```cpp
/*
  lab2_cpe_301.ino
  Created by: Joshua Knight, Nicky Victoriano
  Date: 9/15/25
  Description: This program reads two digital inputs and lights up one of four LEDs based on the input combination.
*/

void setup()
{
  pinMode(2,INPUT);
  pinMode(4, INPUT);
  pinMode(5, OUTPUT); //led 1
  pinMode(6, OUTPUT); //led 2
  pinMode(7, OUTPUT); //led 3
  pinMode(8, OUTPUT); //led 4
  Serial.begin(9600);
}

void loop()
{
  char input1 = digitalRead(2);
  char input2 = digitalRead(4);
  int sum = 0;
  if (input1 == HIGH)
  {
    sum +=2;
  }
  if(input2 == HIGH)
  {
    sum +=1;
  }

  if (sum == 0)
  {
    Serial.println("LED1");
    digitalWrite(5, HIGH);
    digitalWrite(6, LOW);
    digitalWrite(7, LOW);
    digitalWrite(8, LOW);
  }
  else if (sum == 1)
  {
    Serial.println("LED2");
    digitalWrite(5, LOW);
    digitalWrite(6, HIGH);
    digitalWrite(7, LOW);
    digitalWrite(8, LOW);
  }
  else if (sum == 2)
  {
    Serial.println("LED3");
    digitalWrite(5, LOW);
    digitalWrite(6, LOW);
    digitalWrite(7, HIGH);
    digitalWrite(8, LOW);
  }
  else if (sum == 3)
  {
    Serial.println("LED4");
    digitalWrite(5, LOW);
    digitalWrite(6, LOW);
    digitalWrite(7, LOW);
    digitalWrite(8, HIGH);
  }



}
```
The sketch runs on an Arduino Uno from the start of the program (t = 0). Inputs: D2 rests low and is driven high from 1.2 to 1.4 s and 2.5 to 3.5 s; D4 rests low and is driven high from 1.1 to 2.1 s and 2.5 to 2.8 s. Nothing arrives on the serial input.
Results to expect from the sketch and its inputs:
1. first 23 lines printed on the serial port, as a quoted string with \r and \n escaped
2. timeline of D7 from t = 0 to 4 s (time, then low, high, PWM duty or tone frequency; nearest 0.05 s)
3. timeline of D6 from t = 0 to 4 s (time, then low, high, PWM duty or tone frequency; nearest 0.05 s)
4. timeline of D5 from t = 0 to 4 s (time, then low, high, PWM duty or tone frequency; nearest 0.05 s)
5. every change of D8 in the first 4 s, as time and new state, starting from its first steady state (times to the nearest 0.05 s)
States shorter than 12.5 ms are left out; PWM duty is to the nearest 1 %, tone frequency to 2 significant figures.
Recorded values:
"LED1\r\nLED1\r\nLED1\r\nLED1\r\nLED1\r\nLED1\r\nLED1\r\nLED1\r\nLED1\r\nLED1\r\nLED1\r\nLED1\r\nLED1\r\nLED1\r\nLED1\r\nLED1\r\nLED1\r\nLED1\r\nLED1\r\nLED1\r\nLED1\r\nLED1\r\nLED1\r\n"
0 s low; 2.8 s high; 3.5 s low
0 s low; 1.1 s high; 1.2 s low; 1.4 s high; 2.1 s low
0 s high; 1.1 s low; 2.1 s high; 2.5 s low; 3.5 s high
0 s low; 1.2 s high; 1.4 s low; 2.5 s high; 2.8 s low
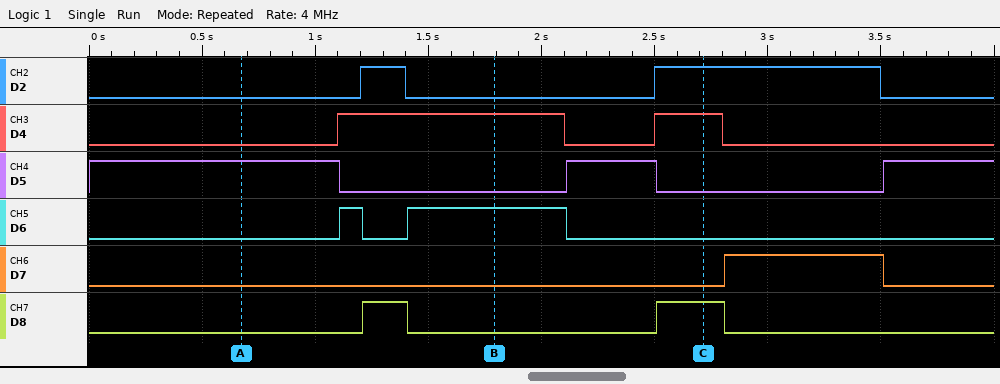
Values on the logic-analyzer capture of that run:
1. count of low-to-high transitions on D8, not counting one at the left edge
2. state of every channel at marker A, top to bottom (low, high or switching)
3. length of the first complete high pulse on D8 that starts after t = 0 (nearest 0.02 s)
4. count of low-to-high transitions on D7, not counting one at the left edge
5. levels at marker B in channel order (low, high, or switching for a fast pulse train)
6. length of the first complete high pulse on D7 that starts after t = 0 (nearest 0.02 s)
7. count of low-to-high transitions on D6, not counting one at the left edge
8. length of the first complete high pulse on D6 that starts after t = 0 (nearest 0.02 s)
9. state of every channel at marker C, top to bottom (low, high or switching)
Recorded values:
2
D2 low, D4 low, D5 high, D6 low, D7 low, D8 low
0.20 s
1
D2 low, D4 high, D5 low, D6 high, D7 low, D8 low
0.70 s
2
0.10 s
D2 high, D4 high, D5 low, D6 low, D7 low, D8 high
